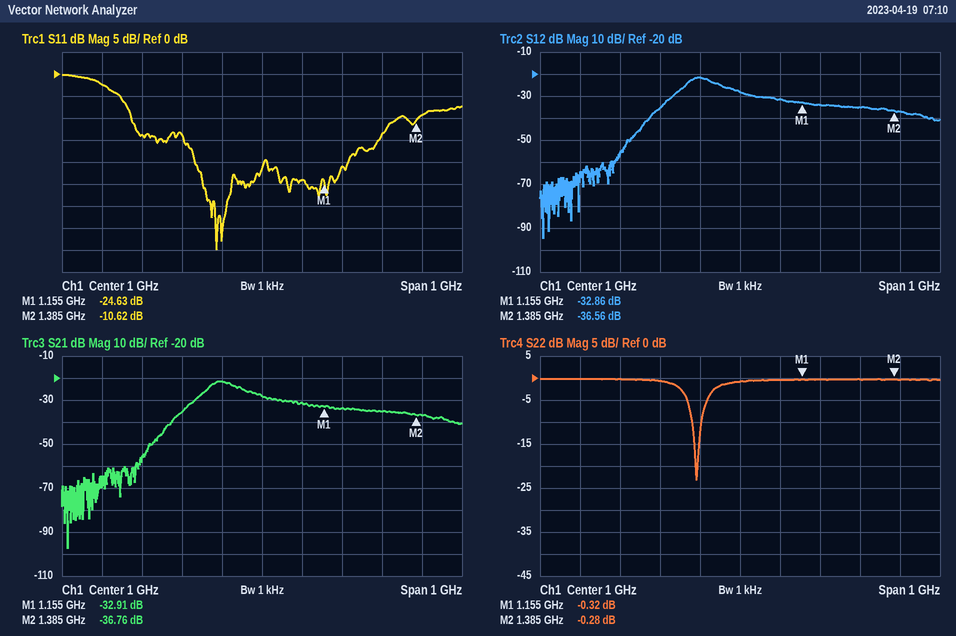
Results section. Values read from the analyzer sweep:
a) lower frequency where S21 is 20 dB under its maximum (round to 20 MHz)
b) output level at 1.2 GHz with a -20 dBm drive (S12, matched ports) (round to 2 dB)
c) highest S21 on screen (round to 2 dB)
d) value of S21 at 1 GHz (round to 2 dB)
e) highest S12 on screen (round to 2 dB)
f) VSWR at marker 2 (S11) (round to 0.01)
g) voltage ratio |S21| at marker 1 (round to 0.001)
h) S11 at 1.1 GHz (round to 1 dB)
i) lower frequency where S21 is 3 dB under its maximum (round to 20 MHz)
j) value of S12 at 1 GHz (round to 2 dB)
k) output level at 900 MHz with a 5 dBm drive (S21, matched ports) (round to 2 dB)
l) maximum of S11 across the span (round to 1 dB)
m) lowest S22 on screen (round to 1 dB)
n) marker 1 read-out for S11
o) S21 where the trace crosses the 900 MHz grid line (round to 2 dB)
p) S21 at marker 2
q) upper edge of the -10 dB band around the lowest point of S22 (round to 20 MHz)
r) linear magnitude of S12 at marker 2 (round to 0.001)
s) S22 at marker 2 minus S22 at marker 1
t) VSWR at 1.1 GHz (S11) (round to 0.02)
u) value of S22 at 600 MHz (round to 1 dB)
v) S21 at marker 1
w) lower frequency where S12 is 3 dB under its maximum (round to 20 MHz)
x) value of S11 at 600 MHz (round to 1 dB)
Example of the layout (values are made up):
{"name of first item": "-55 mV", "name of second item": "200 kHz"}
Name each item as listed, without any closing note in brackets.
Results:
{"lower frequency where S21 is 20 dB under its maximum": "760 MHz", "output level at 1.2 GHz with a -20 dBm drive (S12, matched ports)": "-54 dBm", "highest S21 on screen": "-22 dB", "value of S21 at 1 GHz": "-28 dB", "highest S12 on screen": "-22 dB", "VSWR at marker 2 (S11)": "1.83", "voltage ratio |S21| at marker 1": "0.023", "S11 at 1.1 GHz": "-24 dB", "lower frequency where S21 is 3 dB under its maximum": "860 MHz", "value of S12 at 1 GHz": "-28 dB", "output level at 900 MHz with a 5 dBm drive (S21, matched ports)": "-16 dBm", "maximum of S11 across the span": "0 dB", "lowest S22 on screen": "-23 dB", "marker 1 read-out for S11": "-24.63 dB", "S21 where the trace crosses the 900 MHz grid line": "-22 dB", "S21 at marker 2": "-36.76 dB", "upper edge of the -10 dB band around the lowest point of S22": "900 MHz", "linear magnitude of S12 at marker 2": "0.015", "S22 at marker 2 minus S22 at marker 1": "0.04 dB", "VSWR at 1.1 GHz (S11)": "1.14", "value of S22 at 600 MHz": "0 dB", "S21 at marker 1": "-32.91 dB", "lower frequency where S12 is 3 dB under its maximum": "860 MHz", "value of S11 at 600 MHz": "-2 dB"}
